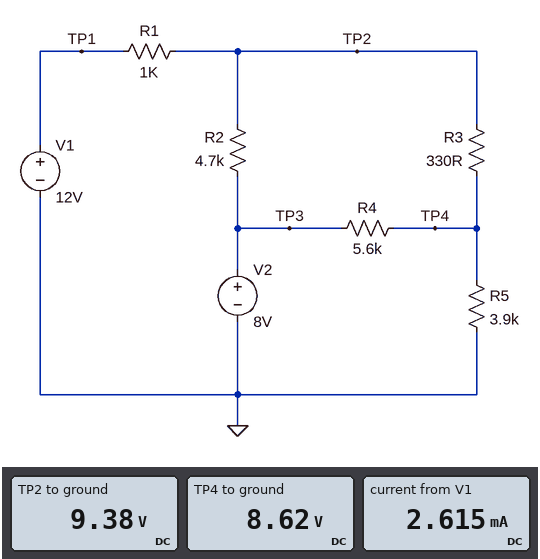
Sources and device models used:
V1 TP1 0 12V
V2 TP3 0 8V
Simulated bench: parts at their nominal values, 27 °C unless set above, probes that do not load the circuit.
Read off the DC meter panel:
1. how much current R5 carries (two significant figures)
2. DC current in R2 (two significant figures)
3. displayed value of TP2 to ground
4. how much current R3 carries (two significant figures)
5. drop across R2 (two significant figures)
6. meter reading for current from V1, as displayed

2.2 mA
290 µA
9.38 V
2.3 mA
1.4 V
2.615 mA
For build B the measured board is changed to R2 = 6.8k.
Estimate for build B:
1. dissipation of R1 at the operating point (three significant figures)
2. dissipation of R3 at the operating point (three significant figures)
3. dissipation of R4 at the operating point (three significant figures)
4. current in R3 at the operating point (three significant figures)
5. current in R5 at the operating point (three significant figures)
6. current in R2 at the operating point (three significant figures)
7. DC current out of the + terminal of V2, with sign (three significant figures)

6.53 mW
1.81 mW
80.4 µW
2.34 mA
2.22 mA
212 µA
-332 µA
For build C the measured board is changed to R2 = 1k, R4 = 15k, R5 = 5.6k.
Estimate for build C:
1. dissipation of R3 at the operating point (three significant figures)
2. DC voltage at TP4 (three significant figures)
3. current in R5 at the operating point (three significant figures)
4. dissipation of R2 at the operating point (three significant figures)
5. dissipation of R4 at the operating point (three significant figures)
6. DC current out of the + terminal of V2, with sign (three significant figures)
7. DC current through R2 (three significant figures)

839 µW
8.68 V
1.55 mA
1.45 mW
30.5 µW
-1.25 mA
1.20 mA
